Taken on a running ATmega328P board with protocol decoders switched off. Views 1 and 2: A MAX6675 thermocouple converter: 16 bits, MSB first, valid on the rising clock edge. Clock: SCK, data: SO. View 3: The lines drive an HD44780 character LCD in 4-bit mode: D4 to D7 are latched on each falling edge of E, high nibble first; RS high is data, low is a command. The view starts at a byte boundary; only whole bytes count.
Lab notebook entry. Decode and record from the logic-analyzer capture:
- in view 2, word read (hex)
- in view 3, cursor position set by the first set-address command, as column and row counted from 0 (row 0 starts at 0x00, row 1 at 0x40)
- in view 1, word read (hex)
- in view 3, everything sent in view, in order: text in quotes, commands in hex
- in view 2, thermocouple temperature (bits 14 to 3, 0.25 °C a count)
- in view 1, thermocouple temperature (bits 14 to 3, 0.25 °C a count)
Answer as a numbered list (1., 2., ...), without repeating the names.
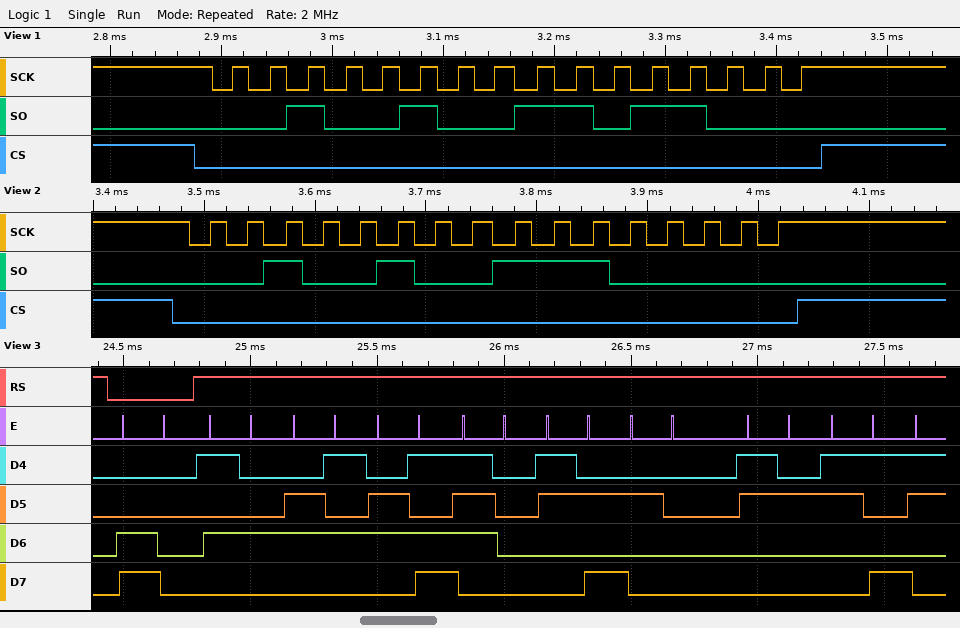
1. 0x24E0
2. column 0, row 1
3. 0x24D8
4. 0xC0 "Temp: 29"
5. 295.00 °C
6. 294.75 °C
